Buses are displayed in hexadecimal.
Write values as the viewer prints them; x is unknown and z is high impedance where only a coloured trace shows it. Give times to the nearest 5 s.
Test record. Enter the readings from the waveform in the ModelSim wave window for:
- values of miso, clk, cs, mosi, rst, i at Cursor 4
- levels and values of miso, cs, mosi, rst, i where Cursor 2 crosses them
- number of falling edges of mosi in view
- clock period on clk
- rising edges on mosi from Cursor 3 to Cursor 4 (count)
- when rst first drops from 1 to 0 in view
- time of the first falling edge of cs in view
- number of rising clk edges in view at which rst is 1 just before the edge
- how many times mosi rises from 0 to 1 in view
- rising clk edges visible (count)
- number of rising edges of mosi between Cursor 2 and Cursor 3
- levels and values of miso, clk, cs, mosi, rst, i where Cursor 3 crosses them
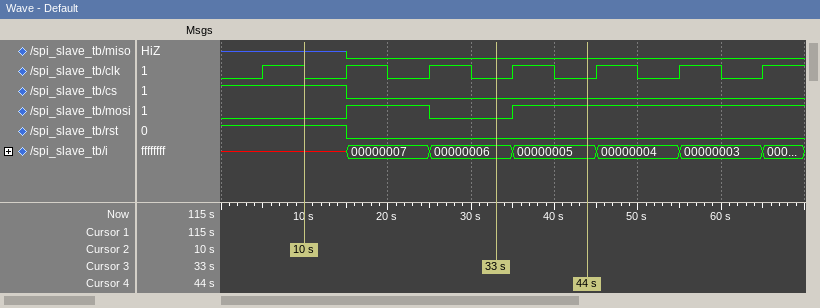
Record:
miso=0, clk=0, cs=0, mosi=1, rst=0, i=00000005
miso=z, cs=1, mosi=0, rst=1, i=x
1
10 s
1
15 s
15 s
2
2
7
1
miso=0, clk=0, cs=0, mosi=0, rst=0, i=00000006
